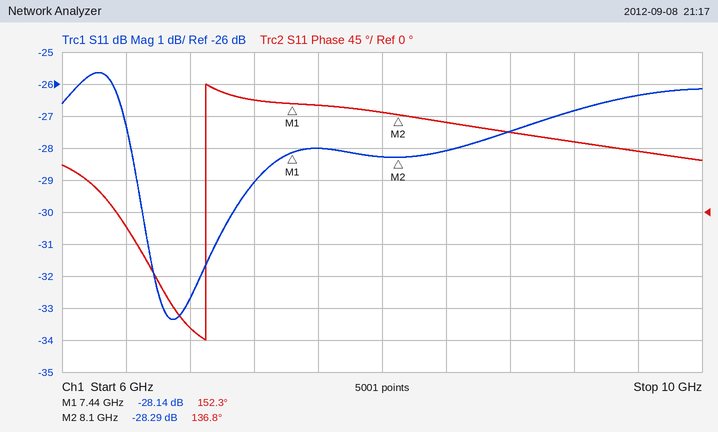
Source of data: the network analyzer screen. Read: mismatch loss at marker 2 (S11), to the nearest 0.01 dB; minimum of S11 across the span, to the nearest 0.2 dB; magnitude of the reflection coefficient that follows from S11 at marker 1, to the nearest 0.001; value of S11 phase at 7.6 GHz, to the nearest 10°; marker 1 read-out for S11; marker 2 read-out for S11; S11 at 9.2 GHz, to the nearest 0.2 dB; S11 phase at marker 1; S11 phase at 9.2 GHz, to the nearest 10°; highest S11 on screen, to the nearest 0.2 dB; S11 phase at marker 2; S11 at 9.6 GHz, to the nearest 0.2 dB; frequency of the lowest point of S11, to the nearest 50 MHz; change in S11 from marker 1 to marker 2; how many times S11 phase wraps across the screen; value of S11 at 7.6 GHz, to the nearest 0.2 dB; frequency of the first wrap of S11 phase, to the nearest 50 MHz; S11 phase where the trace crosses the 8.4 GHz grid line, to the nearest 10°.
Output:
0.01 dB
-33.4 dB
0.039
150°
-28.14 dB
-28.29 dB
-26.8 dB
152.3°
100°
-25.6 dB
136.8°
-26.4 dB
6.70 GHz
-0.15 dB
1
-28.0 dB
6.90 GHz
130°
